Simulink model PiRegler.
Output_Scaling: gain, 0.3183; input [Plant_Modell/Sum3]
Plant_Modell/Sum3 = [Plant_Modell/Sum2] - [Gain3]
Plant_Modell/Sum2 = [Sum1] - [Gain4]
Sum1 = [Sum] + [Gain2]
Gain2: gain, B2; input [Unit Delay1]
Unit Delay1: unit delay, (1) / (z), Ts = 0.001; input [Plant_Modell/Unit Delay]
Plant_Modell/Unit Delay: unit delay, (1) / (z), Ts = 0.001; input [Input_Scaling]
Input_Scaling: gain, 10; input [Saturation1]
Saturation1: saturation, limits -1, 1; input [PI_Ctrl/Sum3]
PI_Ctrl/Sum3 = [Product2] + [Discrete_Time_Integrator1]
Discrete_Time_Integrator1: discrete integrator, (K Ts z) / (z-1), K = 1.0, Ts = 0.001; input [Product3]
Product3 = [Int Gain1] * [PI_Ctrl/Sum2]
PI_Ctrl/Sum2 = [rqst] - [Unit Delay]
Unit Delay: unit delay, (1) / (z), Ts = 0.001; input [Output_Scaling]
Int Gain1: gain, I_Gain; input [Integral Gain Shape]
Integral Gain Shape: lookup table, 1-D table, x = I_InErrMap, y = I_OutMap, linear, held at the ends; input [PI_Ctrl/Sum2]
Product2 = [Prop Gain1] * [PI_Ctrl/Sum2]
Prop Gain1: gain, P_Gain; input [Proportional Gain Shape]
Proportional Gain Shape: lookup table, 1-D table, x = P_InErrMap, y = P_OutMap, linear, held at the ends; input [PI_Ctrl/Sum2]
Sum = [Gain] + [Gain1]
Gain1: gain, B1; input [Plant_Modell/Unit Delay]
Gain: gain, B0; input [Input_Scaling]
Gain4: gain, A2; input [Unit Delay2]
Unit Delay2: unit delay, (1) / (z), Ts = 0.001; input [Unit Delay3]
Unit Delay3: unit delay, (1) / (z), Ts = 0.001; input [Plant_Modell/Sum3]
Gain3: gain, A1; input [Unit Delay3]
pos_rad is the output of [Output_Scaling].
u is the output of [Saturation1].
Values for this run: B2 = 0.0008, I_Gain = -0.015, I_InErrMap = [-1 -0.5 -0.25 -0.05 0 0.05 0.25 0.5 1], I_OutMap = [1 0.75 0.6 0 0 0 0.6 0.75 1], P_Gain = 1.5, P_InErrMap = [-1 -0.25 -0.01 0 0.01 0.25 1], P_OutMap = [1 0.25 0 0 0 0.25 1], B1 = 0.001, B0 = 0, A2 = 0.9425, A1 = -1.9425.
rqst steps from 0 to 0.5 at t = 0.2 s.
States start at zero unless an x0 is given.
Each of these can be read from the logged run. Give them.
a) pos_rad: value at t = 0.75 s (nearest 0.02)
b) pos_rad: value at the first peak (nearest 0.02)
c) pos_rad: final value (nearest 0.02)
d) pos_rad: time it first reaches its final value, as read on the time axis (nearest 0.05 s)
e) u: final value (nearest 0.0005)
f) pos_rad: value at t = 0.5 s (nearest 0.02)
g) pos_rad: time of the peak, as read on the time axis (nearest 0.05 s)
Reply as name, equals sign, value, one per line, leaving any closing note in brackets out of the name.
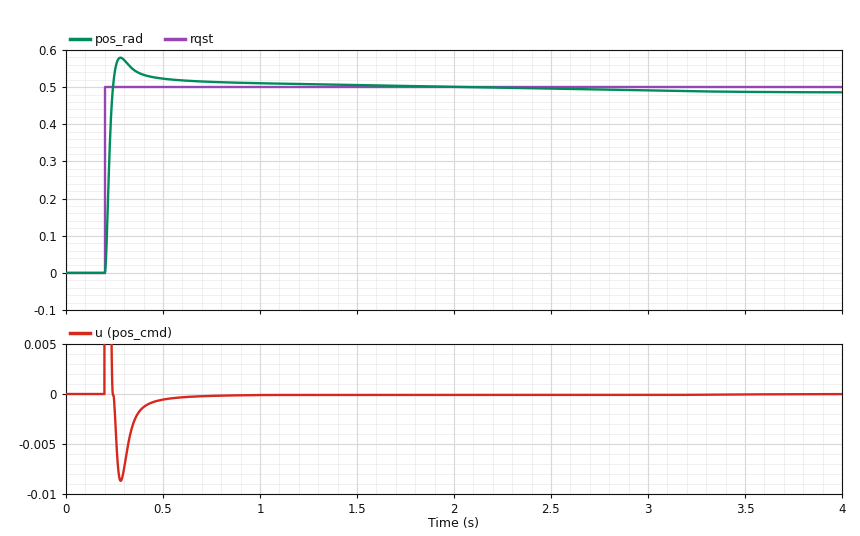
pos_rad: value at t = 0.75 s = 0.52
pos_rad: value at the first peak = 0.58
pos_rad: final value = 0.48
pos_rad: time it first reaches its final value, as read on the time axis = 0.25 s
u: final value = 0.0000
pos_rad: value at t = 0.5 s = 0.52
pos_rad: time of the peak, as read on the time axis = 0.30 s
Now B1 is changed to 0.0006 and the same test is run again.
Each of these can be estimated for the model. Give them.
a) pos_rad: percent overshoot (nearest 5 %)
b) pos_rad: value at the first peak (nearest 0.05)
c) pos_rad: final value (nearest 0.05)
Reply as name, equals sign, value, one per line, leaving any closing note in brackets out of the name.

pos_rad: percent overshoot = 10 %
pos_rad: value at the first peak = 0.55
pos_rad: final value = 0.50
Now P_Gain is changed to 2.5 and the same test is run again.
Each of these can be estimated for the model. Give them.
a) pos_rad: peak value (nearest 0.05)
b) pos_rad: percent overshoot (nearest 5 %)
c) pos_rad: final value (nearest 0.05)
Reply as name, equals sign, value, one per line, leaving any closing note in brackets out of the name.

pos_rad: peak value = 0.65
pos_rad: percent overshoot = 35 %
pos_rad: final value = 0.50
